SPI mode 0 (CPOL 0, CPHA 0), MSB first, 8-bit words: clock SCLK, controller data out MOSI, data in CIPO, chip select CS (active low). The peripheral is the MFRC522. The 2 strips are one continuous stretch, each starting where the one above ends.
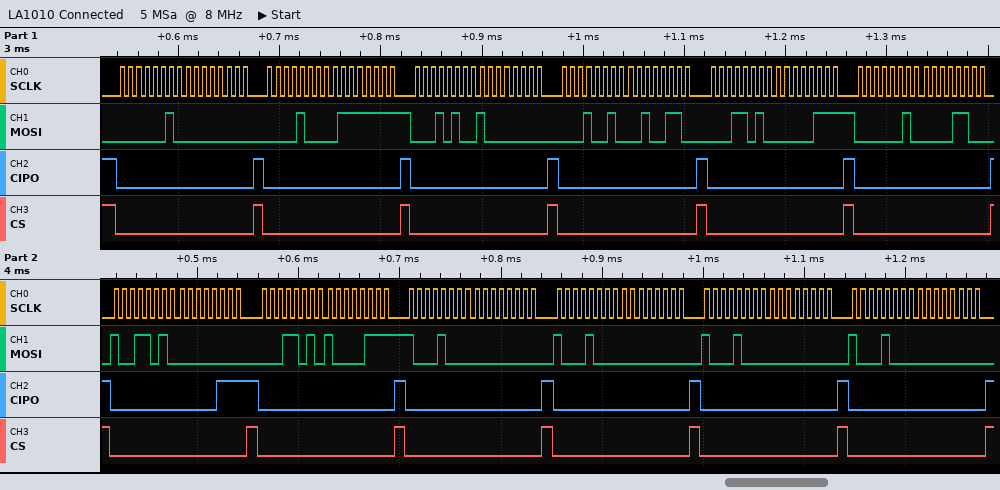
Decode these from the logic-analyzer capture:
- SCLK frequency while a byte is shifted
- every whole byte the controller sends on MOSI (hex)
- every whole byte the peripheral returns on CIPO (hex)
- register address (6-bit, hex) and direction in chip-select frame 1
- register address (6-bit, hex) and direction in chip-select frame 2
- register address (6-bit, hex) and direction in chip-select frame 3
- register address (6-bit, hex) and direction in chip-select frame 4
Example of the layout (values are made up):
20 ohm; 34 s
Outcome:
125 kHz; 02 00 08 7F 14 80 12 26 1A 07 02 0C 9A 00 1A 87 88 00 88 00 88 00 88 00; 00 00 00 00 00 00 00 00 00 00 00 00 00 07 00 00 00 00 00 00 00 00 00 00; 0x01 write; 0x04 write; 0x0A write; 0x09 write
